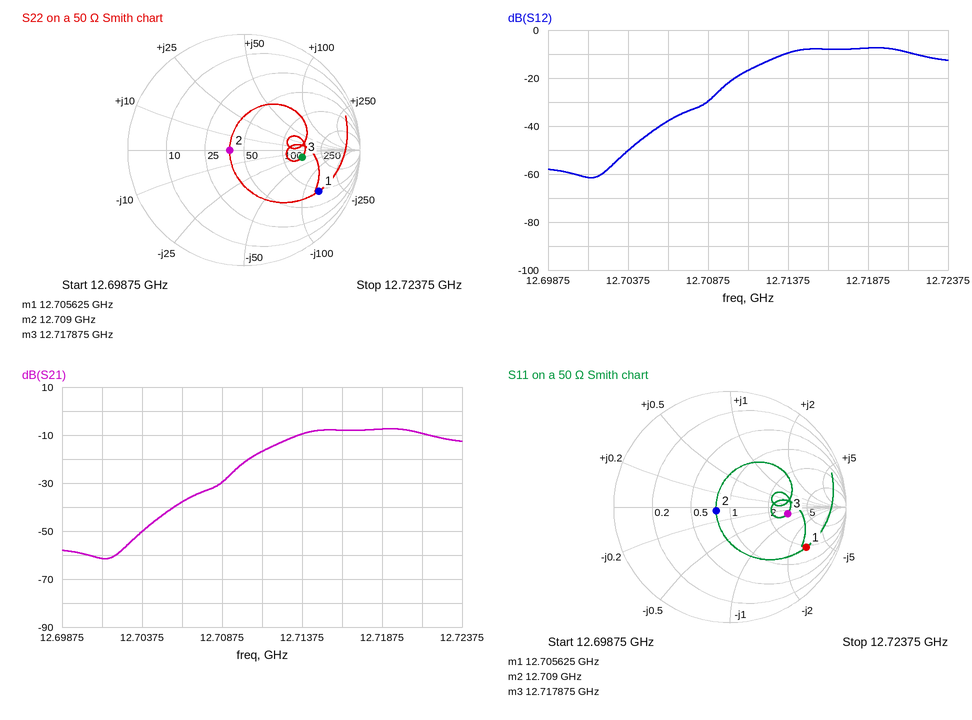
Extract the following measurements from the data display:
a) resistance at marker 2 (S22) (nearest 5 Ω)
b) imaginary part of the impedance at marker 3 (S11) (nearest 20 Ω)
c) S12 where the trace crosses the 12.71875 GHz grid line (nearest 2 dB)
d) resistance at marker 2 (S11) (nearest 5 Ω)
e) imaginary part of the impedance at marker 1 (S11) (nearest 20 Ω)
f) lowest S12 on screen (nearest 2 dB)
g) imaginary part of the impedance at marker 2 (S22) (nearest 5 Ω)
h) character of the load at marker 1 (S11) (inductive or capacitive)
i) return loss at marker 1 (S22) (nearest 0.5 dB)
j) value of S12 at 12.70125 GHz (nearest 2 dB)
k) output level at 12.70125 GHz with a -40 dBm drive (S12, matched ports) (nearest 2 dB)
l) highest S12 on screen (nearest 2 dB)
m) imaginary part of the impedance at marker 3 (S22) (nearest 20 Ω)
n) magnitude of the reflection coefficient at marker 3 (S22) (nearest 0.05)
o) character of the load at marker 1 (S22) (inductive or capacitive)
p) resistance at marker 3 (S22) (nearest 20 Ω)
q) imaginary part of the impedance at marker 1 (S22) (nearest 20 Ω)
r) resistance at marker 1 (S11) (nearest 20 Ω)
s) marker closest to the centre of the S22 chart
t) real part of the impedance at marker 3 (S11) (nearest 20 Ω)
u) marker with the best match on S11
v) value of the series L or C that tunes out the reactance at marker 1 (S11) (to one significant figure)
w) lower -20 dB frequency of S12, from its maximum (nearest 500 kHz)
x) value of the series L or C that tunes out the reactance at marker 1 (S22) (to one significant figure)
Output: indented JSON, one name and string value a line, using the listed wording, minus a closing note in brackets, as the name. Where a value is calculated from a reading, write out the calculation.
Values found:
{
  "resistance at marker 2 (S22)": "40 Ω",
  "imaginary part of the impedance at marker 3 (S11)": "-20 Ω",
  "S12 where the trace crosses the 12.71875 GHz grid line": "-8 dB",
  "resistance at marker 2 (S11)": "40 Ω",
  "imaginary part of the impedance at marker 1 (S11)": "-140 Ω",
  "lowest S12 on screen": "-62 dB",
  "imaginary part of the impedance at marker 2 (S22)": "0 Ω",
  "character of the load at marker 1 (S11)": "capacitive",
  "return loss at marker 1 (S22)": "2.5 dB",
  "value of S12 at 12.70125 GHz": "-62 dB",
  "output level at 12.70125 GHz with a -40 dBm drive (S12, matched ports)": "-40 dBm + (-62 dB) = -102 dBm",
  "highest S12 on screen": "-8 dB",
  "imaginary part of the impedance at marker 3 (S22)": "-20 Ω",
  "magnitude of the reflection coefficient at marker 3 (S22)": "0.50",
  "character of the load at marker 1 (S22)": "capacitive",
  "resistance at marker 3 (S22)": "140 Ω",
  "imaginary part of the impedance at marker 1 (S22)": "-140 Ω",
  "resistance at marker 1 (S11)": "100 Ω",
  "marker closest to the centre of the S22 chart": "marker 2",
  "real part of the impedance at marker 3 (S11)": "140 Ω",
  "marker with the best match on S11": "marker 2",
  "value of the series L or C that tunes out the reactance at marker 1 (S11)": "L = 140 Ω/(2π × 12.705625 GHz) ≈ 2 nH",
  "lower -20 dB frequency of S12, from its maximum": "12.7090 GHz",
  "value of the series L or C that tunes out the reactance at marker 1 (S22)": "L = 140 Ω/(2π × 12.705625 GHz) ≈ 2 nH"
}
